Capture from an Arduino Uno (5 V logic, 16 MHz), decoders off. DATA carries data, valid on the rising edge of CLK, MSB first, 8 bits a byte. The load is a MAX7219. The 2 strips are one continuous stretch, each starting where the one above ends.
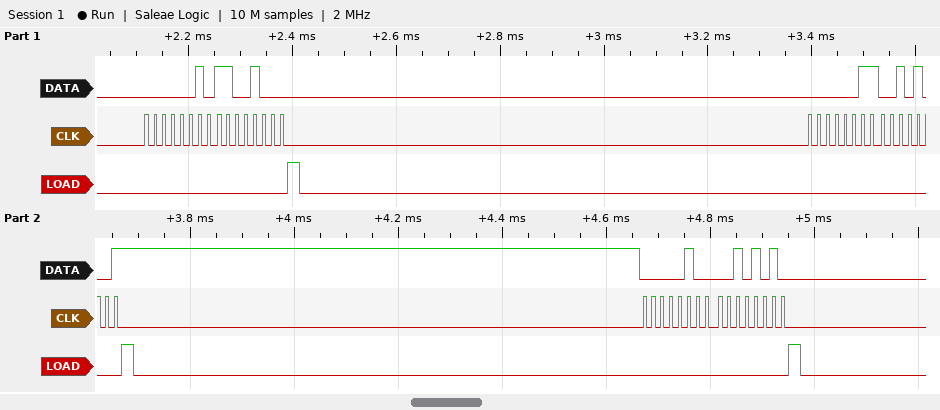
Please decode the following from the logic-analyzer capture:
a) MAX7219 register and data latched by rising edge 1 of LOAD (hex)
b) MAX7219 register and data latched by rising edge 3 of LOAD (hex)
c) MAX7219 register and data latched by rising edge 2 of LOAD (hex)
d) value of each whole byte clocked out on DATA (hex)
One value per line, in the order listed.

register 0x2, data 0xC8
register 0x4, data 0x2A
register 0x3, data 0x29
02 C8 03 29 04 2A
